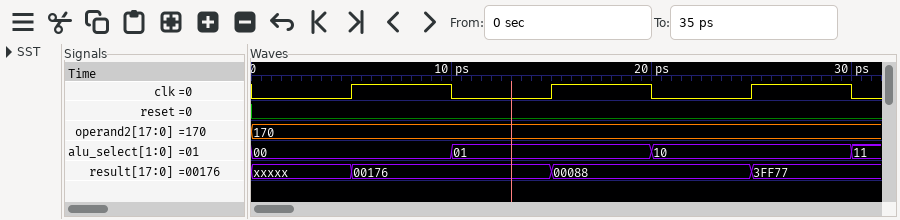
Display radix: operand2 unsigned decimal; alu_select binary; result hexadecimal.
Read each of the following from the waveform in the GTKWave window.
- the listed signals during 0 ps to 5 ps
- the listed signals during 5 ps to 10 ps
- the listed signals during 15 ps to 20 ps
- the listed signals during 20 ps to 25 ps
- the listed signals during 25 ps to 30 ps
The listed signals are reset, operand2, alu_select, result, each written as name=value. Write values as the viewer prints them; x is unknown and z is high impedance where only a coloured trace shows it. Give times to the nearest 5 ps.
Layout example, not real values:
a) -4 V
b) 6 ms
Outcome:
a) reset=0, operand2=170, alu_select=00, result=xxxxx
b) reset=0, operand2=170, alu_select=00, result=00176
c) reset=0, operand2=170, alu_select=01, result=00088
d) reset=0, operand2=170, alu_select=10, result=00088
e) reset=0, operand2=170, alu_select=10, result=3FF77
